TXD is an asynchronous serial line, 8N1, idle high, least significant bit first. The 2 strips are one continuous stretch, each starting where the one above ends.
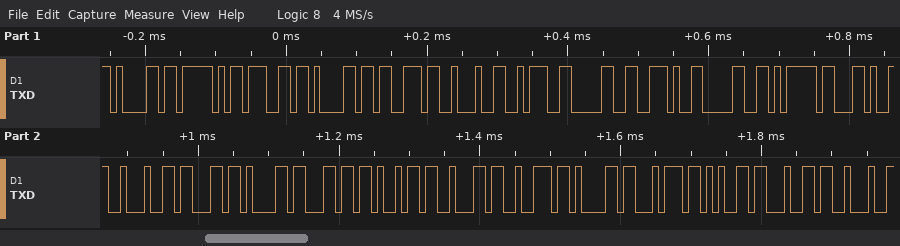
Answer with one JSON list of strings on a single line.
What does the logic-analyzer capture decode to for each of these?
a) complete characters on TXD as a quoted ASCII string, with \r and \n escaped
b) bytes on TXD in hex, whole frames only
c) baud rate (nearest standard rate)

["\"a_gas\\\":0.0},\\\"calibrated\\\"\"", "0x61 0x5F 0x67 0x61 0x73 0x22 0x3A 0x30 0x2E 0x30 0x7D 0x2C 0x22 0x63 0x61 0x6C 0x69 0x62 0x72 0x61 0x74 0x65 0x64 0x22", "115200 baud"]
